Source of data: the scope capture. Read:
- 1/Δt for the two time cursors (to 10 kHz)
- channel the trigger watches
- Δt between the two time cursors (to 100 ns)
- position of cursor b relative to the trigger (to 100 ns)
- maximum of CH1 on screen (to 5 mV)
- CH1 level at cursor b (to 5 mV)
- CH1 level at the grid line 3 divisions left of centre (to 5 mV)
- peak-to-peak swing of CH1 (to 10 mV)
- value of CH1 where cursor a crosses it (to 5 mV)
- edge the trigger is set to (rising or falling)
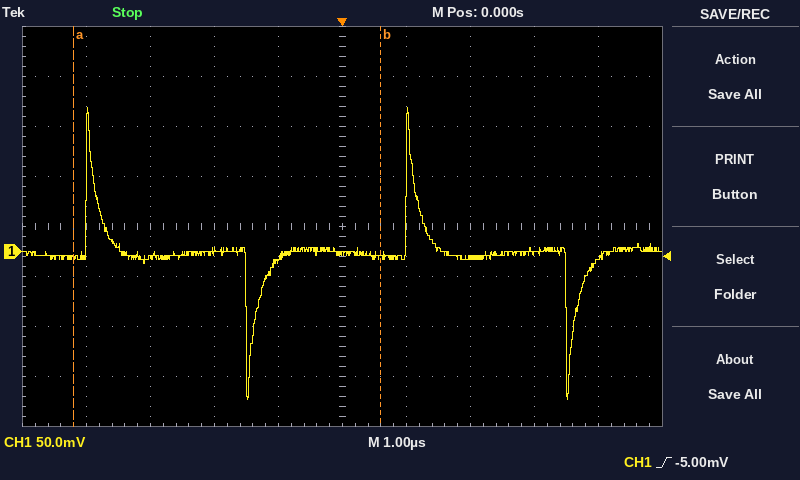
210 kHz
CH1
4.8 µs
+600 ns
145 mV
-5 mV
-5 mV
290 mV
-5 mV
rising
